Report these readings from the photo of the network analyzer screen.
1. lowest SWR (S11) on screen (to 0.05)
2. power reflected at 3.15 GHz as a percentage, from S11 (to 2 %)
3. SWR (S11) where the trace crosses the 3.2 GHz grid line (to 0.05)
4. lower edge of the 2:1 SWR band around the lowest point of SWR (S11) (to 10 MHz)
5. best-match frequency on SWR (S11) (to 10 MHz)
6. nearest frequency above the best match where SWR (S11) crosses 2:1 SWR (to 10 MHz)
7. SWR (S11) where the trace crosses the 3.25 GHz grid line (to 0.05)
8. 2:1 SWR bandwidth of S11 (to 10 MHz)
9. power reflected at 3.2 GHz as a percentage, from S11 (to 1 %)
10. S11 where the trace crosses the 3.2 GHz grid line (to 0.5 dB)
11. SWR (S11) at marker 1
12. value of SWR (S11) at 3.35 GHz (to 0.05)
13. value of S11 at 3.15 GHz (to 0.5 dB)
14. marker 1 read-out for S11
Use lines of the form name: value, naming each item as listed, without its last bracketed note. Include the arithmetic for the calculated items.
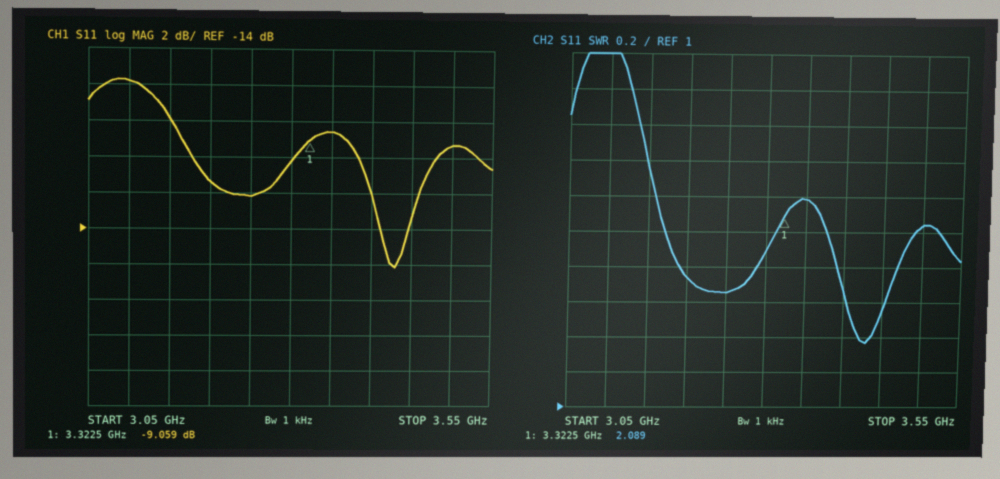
lowest SWR (S11) on screen: 1.35
power reflected at 3.15 GHz as a percentage, from S11: 10^(-8/10) ≈ 16 %
SWR (S11) where the trace crosses the 3.2 GHz grid line: 1.75
lower edge of the 2:1 SWR band around the lowest point of SWR (S11): 3.38 GHz
best-match frequency on SWR (S11): 3.43 GHz
nearest frequency above the best match where SWR (S11) crosses 2:1 SWR: 3.49 GHz
SWR (S11) where the trace crosses the 3.25 GHz grid line: 1.65
2:1 SWR bandwidth of S11: 3.49 GHz − 3.38 GHz = 110 MHz
power reflected at 3.2 GHz as a percentage, from S11: 10^(-11.5/10) ≈ 7 %
S11 where the trace crosses the 3.2 GHz grid line: -11.5 dB
SWR (S11) at marker 1: 2.089
value of SWR (S11) at 3.35 GHz: 2.20
value of S11 at 3.15 GHz: -8.0 dB
marker 1 read-out for S11: -9.059 dB
